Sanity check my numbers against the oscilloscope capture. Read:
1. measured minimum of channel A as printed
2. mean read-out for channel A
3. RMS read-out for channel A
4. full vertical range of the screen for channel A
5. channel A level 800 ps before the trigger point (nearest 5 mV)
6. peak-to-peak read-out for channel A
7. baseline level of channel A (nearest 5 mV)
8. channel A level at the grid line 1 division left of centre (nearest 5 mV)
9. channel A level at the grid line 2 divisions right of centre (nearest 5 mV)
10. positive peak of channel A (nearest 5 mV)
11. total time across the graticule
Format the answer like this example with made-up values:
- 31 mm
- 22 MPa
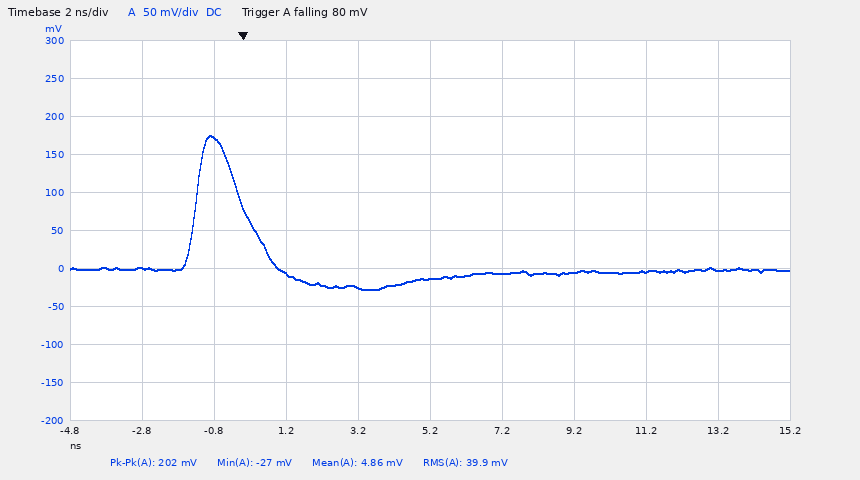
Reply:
- -27 mV
- 4.86 mV
- 39.9 mV
- 500 mV
- 170 mV
- 202 mV
- -5 mV
- -25 mV
- -5 mV
- 175 mV
- 20 ns
